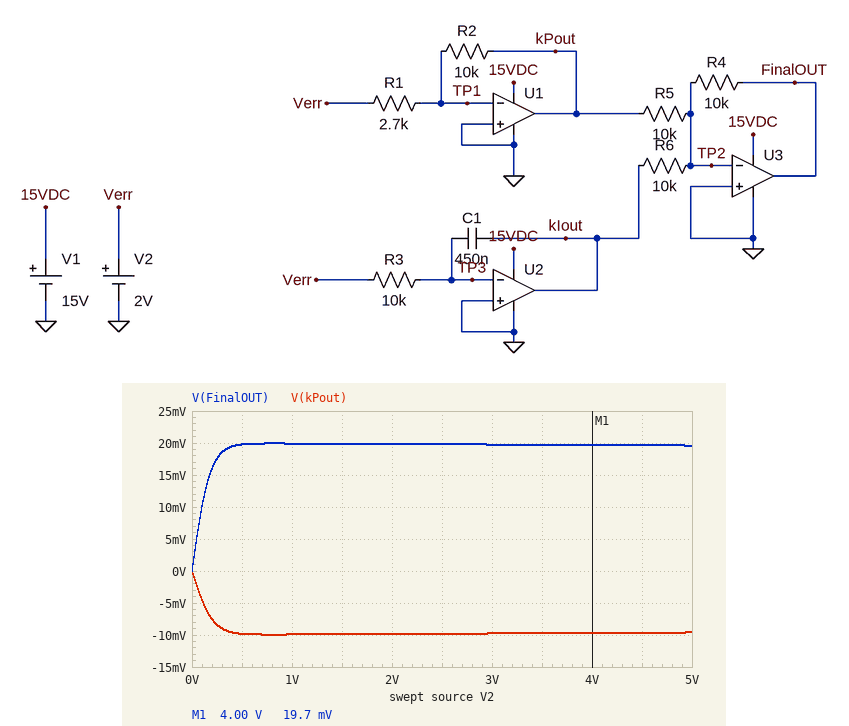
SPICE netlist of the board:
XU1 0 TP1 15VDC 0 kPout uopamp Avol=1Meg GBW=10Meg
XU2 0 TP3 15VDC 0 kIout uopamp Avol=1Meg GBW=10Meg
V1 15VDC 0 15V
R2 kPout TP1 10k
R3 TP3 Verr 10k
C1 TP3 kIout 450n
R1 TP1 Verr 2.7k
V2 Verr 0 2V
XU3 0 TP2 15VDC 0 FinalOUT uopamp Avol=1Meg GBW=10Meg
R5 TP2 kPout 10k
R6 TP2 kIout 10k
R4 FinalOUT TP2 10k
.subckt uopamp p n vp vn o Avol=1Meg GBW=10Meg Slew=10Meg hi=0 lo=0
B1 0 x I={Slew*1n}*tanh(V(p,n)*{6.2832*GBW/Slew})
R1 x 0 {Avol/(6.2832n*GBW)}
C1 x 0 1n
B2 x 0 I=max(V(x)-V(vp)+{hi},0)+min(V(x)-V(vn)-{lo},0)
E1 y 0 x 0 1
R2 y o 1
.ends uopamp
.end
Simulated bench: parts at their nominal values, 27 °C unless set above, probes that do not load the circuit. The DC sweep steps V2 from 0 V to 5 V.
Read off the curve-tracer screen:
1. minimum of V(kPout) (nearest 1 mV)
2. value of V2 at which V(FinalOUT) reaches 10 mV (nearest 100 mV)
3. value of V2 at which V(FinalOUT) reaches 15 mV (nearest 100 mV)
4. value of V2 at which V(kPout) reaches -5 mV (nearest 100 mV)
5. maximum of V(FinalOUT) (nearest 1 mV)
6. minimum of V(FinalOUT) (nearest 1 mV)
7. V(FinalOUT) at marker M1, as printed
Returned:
-10 mV
100 mV
200 mV
100 mV
20 mV
0 V
19.7 mV
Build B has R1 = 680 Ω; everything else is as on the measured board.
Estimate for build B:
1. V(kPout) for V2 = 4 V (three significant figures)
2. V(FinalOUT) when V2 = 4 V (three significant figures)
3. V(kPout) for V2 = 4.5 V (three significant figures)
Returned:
-9.62 mV
19.6 mV
-9.58 mV
